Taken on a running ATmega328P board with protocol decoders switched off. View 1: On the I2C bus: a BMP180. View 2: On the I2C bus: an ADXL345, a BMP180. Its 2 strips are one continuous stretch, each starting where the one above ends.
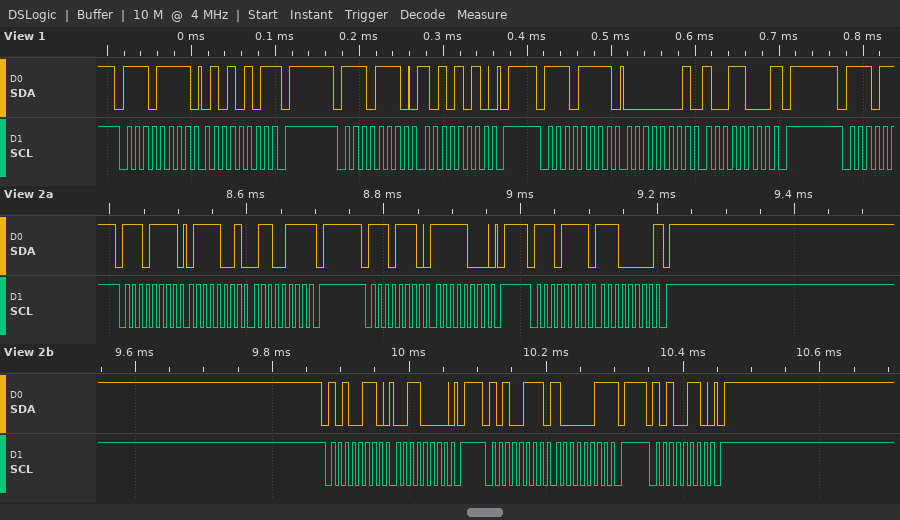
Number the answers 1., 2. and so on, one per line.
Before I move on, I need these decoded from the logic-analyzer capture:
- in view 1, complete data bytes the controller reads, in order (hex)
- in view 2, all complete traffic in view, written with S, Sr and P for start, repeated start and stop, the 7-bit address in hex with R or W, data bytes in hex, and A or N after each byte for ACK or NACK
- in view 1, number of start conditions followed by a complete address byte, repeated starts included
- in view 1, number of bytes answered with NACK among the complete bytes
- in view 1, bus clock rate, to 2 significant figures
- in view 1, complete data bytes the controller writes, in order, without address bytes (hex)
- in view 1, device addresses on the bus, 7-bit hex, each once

1. 55 01 98
2. S 77R A 79 A 67 N P S 77W A F8 A P S 77R A E0 N P S 53W A 30 A P S 53R A 83 N P S 53W A P
3. 3
4. 2
5. 100 kHz
6. AA
7. 0x77
